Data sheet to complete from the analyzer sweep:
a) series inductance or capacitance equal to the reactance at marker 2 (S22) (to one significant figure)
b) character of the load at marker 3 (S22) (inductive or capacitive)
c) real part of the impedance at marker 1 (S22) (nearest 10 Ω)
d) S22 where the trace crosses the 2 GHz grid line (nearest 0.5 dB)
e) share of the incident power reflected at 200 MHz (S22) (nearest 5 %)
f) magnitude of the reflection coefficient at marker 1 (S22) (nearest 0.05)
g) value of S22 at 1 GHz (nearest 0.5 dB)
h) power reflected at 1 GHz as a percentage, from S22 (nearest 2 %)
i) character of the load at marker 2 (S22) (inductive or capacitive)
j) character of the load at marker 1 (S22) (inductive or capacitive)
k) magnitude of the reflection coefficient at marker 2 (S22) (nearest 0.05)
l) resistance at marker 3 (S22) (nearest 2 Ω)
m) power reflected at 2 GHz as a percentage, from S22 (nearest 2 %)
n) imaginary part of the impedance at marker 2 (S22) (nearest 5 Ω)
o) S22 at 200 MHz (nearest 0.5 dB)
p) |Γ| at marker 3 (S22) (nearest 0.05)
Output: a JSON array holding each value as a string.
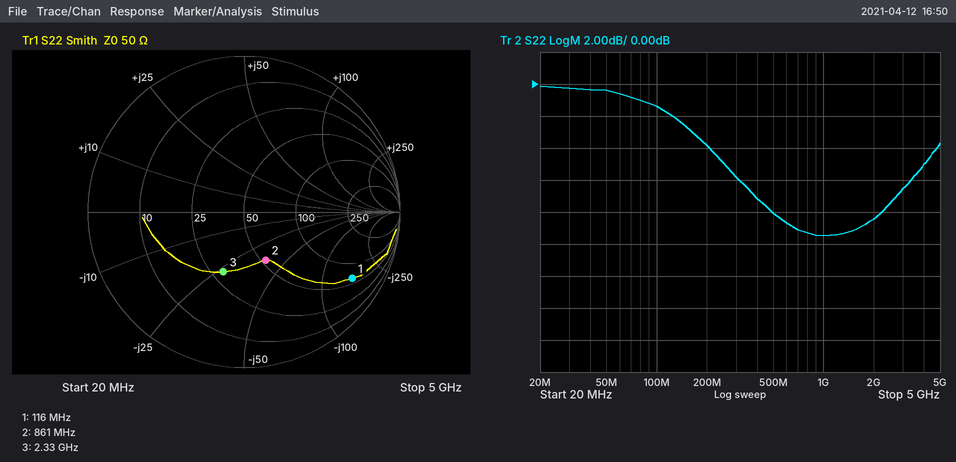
["5 pF", "capacitive", "60 Ω", "-8.5 dB", "40 %", "0.80", "-9.5 dB", "12 %", "capacitive", "capacitive", "0.35", "30 Ω", "14 %", "-35 Ω", "-4.0 dB", "0.40"]
